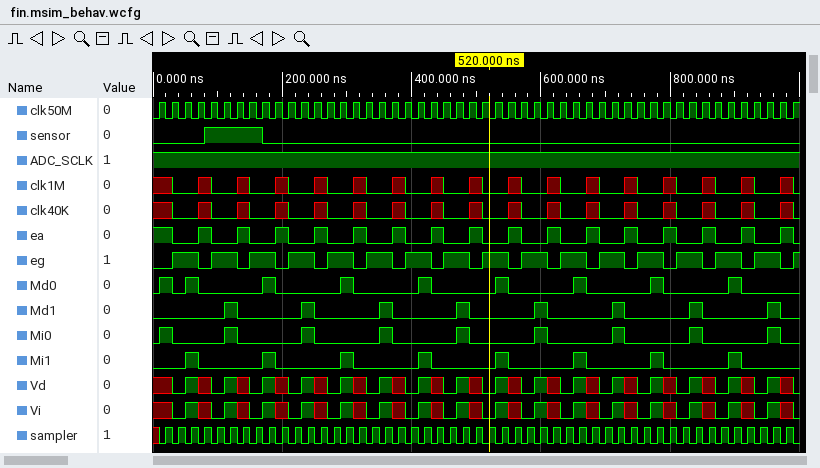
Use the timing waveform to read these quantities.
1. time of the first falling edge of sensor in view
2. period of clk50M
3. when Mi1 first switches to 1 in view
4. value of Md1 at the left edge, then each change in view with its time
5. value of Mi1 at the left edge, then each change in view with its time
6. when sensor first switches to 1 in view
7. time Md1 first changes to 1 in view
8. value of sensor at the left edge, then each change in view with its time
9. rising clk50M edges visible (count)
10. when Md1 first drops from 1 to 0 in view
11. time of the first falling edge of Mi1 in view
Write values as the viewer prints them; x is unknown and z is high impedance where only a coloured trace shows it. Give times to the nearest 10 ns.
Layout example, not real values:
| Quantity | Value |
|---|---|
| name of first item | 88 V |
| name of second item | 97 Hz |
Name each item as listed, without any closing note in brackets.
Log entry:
| Quantity | Value |
|---|---|
| time of the first falling edge of sensor in view | 170 ns |
| period of clk50M | 20 ns |
| when Mi1 first switches to 1 in view | 50 ns |
| value of Md1 at the left edge, then each change in view with its time | 0, 1 at 110 ns, 0 at 130 ns, 1 at 230 ns, 0 at 250 ns, 1 at 350 ns, 0 at 370 ns, 1 at 470 ns, 0 at 490 ns, 1 at 590 ns, 0 at 610 ns, 1 at 710 ns, 0 at 730 ns, 1 at 830 ns, 0 at 850 ns, 1 at 950 ns, 0 at 970 ns |
| value of Mi1 at the left edge, then each change in view with its time | 0, 1 at 50 ns, 0 at 70 ns, 1 at 170 ns, 0 at 190 ns, 1 at 290 ns, 0 at 310 ns, 1 at 410 ns, 0 at 430 ns, 1 at 530 ns, 0 at 550 ns, 1 at 650 ns, 0 at 670 ns, 1 at 770 ns, 0 at 790 ns, 1 at 890 ns, 0 at 910 ns |
| when sensor first switches to 1 in view | 80 ns |
| time Md1 first changes to 1 in view | 110 ns |
| value of sensor at the left edge, then each change in view with its time | 0, 1 at 80 ns, 0 at 170 ns |
| rising clk50M edges visible | 50 |
| when Md1 first drops from 1 to 0 in view | 130 ns |
| time of the first falling edge of Mi1 in view | 70 ns |
